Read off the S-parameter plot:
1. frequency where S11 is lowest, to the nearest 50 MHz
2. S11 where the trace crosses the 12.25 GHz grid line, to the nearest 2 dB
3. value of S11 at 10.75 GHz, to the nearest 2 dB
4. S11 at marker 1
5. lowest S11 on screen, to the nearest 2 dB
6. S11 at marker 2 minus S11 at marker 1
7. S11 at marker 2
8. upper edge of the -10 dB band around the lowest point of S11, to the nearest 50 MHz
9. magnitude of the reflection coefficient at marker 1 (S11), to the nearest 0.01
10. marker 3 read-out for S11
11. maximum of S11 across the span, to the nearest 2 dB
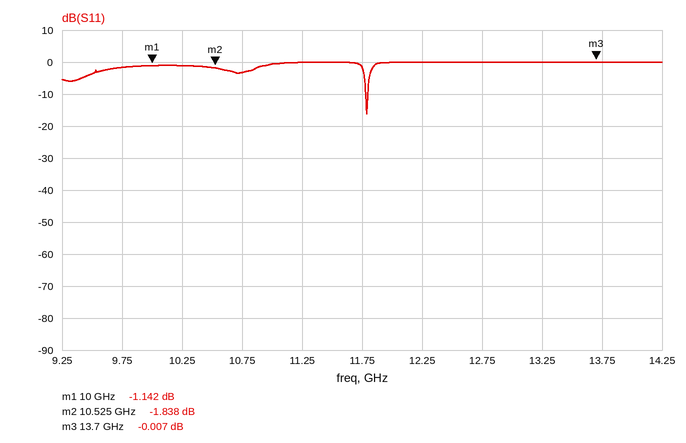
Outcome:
11.80 GHz
0 dB
-4 dB
-1.142 dB
-16 dB
-0.696 dB
-1.838 dB
11.80 GHz
0.88
-0.007 dB
0 dB
